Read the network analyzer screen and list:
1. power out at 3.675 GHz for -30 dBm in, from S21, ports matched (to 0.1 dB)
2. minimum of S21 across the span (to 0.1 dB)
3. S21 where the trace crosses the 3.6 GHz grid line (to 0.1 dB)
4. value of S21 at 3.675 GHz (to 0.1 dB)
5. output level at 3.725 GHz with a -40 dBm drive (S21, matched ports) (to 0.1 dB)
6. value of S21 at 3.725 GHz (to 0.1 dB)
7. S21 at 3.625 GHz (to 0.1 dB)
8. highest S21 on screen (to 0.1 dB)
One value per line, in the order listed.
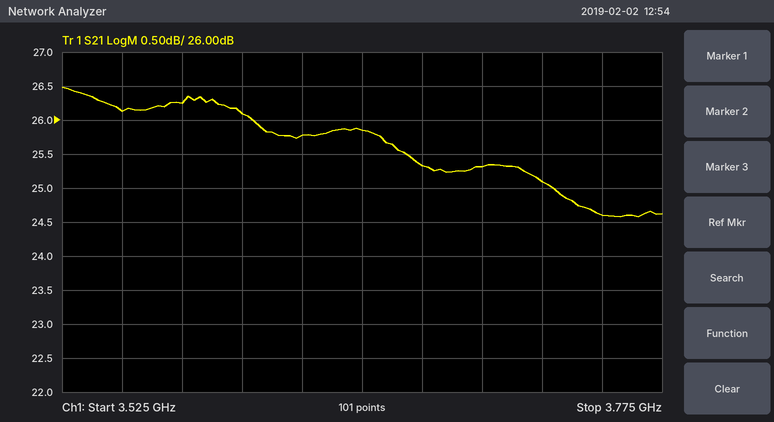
-4.7 dBm
24.6 dB
26.1 dB
25.3 dB
-14.9 dBm
25.1 dB
25.8 dB
26.5 dB
